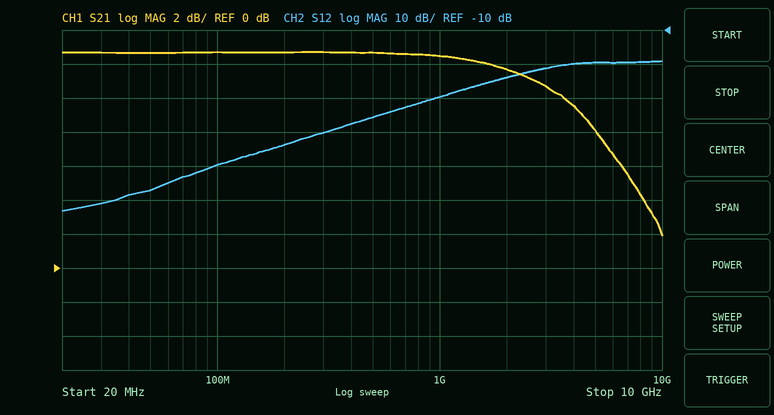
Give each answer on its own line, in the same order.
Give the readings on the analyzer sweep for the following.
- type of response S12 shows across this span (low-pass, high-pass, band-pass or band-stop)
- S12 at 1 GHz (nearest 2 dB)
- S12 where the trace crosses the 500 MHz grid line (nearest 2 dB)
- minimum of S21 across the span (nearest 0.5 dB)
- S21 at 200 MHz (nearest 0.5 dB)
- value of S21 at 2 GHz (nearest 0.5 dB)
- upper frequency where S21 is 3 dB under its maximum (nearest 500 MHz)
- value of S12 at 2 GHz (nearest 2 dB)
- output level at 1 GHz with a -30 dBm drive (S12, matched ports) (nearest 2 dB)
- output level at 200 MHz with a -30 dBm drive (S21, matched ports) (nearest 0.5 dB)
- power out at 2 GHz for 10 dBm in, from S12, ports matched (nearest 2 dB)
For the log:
high-pass
-30 dB
-36 dB
2.0 dB
12.5 dB
11.5 dB
4.0 GHz
-24 dB
-60 dBm
-17.5 dBm
-14 dBm
